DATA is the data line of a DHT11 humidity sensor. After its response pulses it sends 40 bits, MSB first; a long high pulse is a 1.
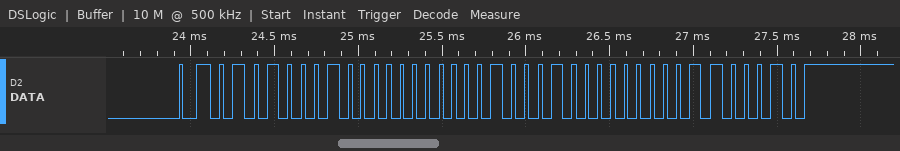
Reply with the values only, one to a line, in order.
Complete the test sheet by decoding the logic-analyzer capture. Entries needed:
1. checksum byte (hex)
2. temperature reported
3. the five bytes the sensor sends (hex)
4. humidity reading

0x62
17.0 °C
51 00 11 00 62
81 %
